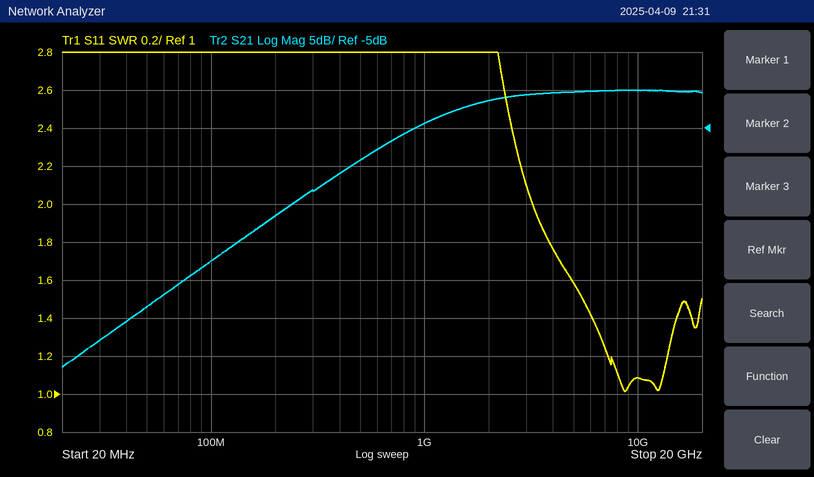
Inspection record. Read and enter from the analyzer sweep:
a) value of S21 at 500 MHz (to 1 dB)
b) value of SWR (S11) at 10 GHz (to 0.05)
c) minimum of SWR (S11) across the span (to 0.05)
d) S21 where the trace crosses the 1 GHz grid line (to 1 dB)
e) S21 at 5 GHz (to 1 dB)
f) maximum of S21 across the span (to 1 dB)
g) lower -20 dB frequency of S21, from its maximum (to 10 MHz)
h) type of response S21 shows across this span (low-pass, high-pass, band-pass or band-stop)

-9 dB
1.10
1.00
-4 dB
0 dB
0 dB
130 MHz
high-pass
